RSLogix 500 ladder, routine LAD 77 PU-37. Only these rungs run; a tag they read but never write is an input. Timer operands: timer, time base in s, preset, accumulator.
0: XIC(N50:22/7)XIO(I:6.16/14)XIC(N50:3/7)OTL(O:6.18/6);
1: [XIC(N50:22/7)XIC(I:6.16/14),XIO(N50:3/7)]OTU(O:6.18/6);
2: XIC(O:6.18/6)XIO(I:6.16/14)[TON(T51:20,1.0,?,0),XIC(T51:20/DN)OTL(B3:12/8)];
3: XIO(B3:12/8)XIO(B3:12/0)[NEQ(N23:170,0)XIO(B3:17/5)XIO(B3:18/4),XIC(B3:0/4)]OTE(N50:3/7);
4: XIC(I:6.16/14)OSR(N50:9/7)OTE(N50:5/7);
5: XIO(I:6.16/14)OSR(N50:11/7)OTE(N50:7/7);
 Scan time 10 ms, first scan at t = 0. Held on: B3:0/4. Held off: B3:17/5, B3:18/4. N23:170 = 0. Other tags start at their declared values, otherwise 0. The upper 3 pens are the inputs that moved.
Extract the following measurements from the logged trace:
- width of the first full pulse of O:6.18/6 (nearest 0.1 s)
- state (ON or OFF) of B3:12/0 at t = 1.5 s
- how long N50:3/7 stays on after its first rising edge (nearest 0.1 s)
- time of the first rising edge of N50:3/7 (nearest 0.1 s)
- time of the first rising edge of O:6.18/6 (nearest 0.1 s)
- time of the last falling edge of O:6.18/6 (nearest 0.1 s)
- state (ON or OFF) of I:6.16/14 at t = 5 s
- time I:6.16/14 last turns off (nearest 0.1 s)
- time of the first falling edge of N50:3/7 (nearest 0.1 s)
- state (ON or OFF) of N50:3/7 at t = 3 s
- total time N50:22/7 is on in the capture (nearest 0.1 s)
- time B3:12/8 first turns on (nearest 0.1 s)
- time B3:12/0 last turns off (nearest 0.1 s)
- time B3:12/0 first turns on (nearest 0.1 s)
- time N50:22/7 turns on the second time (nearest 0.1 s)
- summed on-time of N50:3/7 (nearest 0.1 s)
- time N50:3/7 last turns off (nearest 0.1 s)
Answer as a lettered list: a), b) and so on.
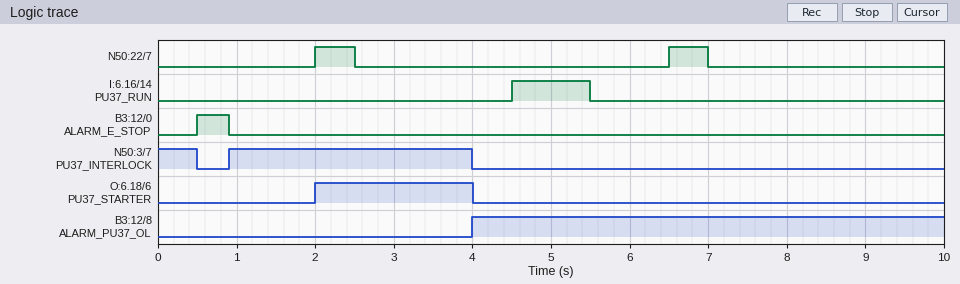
a) 2.0 s
b) OFF
c) 3.1 s
d) 0.9 s
e) 2.0 s
f) 4.0 s
g) ON
h) 5.5 s
i) 0.5 s
j) ON
k) 1.0 s
l) 4.0 s
m) 0.9 s
n) 0.5 s
o) 6.5 s
p) 3.6 s
q) 4.0 s
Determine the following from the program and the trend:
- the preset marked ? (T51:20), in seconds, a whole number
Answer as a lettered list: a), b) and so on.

a) 2 s
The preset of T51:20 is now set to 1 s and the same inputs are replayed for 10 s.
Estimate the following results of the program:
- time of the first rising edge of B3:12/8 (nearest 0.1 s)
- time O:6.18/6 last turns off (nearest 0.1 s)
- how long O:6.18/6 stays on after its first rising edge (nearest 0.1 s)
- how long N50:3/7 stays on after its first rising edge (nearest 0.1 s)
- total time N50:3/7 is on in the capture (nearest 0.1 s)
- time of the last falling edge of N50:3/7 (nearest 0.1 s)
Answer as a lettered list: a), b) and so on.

a) 3.0 s
b) 3.0 s
c) 1.0 s
d) 2.1 s
e) 2.6 s
f) 3.0 s
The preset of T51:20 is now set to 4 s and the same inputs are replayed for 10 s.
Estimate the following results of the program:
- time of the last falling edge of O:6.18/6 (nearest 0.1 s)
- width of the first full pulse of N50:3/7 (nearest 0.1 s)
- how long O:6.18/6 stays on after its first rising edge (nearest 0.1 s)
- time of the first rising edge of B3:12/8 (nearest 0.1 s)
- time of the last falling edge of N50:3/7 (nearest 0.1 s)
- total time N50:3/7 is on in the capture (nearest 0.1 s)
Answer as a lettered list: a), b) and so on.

a) 9.5 s
b) 8.6 s
c) 7.5 s
d) 9.5 s
e) 9.5 s
f) 9.1 s
